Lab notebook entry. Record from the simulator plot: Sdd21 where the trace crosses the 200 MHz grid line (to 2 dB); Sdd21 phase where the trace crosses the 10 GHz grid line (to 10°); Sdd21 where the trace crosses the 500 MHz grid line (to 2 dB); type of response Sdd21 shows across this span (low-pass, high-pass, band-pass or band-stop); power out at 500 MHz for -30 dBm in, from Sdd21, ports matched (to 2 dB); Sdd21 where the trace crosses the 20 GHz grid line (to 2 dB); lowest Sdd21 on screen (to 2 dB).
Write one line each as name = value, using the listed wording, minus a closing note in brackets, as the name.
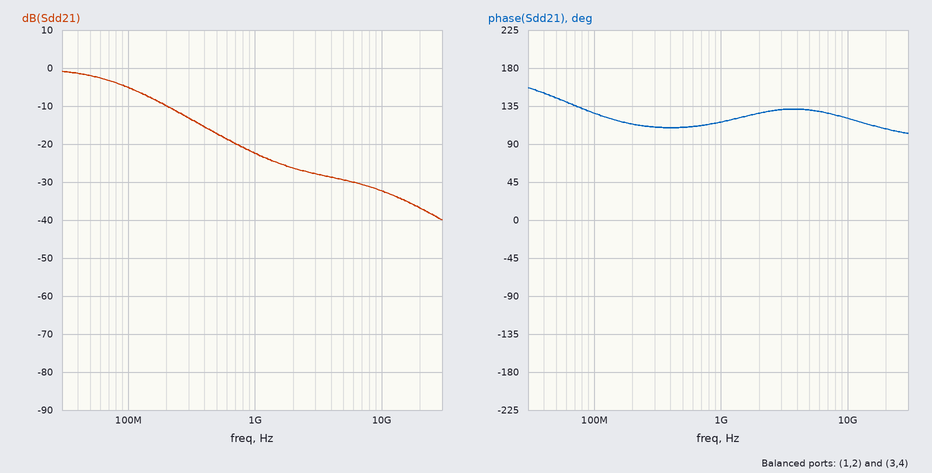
Sdd21 where the trace crosses the 200 MHz grid line = -10 dB
Sdd21 phase where the trace crosses the 10 GHz grid line = 120°
Sdd21 where the trace crosses the 500 MHz grid line = -18 dB
type of response Sdd21 shows across this span = low-pass
power out at 500 MHz for -30 dBm in, from Sdd21, ports matched = -48 dBm
Sdd21 where the trace crosses the 20 GHz grid line = -36 dB
lowest Sdd21 on screen = -40 dB
